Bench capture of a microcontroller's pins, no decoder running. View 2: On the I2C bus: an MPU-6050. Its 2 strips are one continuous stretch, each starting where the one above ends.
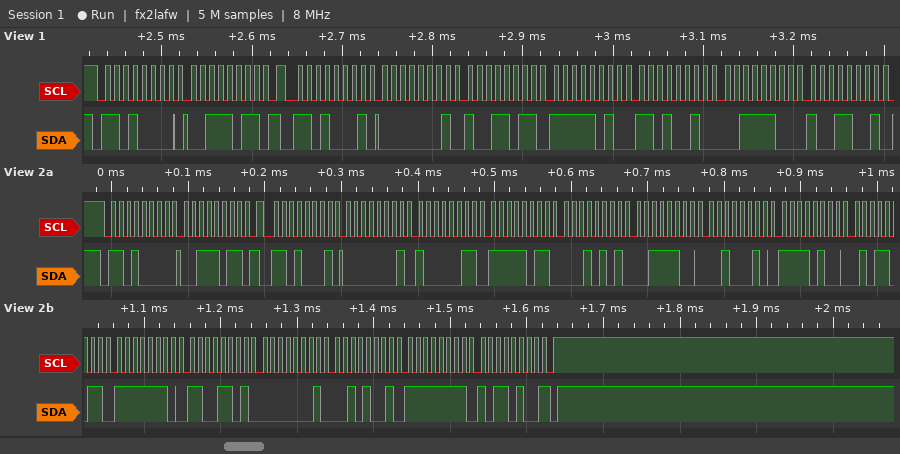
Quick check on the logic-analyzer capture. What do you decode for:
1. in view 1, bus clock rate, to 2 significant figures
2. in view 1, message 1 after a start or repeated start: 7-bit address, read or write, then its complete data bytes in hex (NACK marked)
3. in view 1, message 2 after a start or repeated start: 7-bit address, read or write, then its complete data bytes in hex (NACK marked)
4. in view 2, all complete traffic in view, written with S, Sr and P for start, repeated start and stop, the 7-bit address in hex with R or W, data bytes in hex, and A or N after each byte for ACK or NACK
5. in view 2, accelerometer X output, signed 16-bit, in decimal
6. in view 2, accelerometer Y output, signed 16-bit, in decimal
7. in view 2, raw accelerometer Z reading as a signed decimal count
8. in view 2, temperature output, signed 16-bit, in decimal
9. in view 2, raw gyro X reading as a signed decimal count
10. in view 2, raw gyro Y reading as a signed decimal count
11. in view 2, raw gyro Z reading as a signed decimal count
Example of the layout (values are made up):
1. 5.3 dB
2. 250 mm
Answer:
1. 100 kHz
2. 0x68 write: 3B
3. 0x68 read: 01 9B FA D2 3C 99
4. S 68W A 3B A Sr 68R A 01 A 83 A FB A 15 A 3C A 22 A F4 A 5B A FE A CD A 01 A 29 A FF A B4 N P
5. 387
6. -1259
7. 15394
8. -2981
9. -307
10. 297
11. -76
